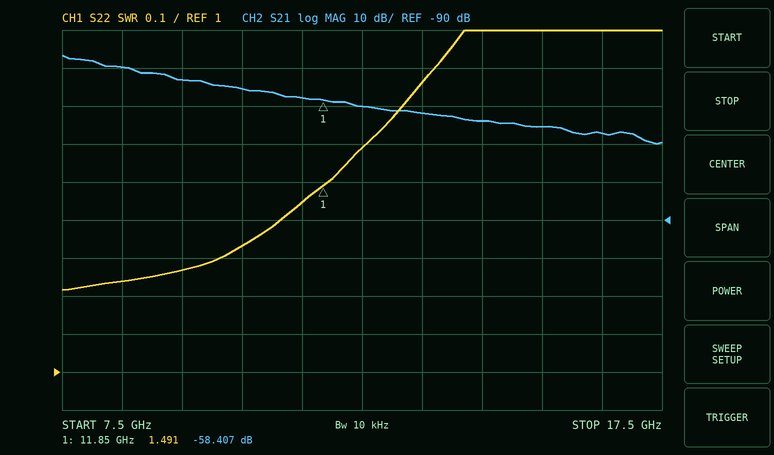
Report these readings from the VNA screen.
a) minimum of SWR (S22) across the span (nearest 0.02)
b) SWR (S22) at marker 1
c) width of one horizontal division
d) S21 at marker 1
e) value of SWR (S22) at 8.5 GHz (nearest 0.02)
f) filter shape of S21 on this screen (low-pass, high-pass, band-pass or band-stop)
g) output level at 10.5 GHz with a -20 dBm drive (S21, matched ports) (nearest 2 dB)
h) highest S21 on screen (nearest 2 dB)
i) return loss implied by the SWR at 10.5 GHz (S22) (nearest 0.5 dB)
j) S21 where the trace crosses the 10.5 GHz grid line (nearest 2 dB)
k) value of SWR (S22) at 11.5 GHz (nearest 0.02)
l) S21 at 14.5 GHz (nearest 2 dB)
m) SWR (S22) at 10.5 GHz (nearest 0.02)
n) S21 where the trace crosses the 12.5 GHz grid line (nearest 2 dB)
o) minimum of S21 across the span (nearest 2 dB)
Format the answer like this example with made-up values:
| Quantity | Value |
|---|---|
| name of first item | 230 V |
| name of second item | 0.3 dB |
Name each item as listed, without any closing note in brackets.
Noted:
| Quantity | Value |
|---|---|
| minimum of SWR (S22) across the span | 1.22 |
| SWR (S22) at marker 1 | 1.491 |
| width of one horizontal division | 1 GHz |
| S21 at marker 1 | -58.407 dB |
| value of SWR (S22) at 8.5 GHz | 1.24 |
| filter shape of S21 on this screen | low-pass |
| output level at 10.5 GHz with a -20 dBm drive (S21, matched ports) | -76 dBm |
| highest S21 on screen | -46 dB |
| return loss implied by the SWR at 10.5 GHz (S22) | 17.0 dB |
| S21 where the trace crosses the 10.5 GHz grid line | -56 dB |
| value of SWR (S22) at 11.5 GHz | 1.44 |
| S21 at 14.5 GHz | -64 dB |
| SWR (S22) at 10.5 GHz | 1.34 |
| S21 where the trace crosses the 12.5 GHz grid line | -60 dB |
| minimum of S21 across the span | -70 dB |
